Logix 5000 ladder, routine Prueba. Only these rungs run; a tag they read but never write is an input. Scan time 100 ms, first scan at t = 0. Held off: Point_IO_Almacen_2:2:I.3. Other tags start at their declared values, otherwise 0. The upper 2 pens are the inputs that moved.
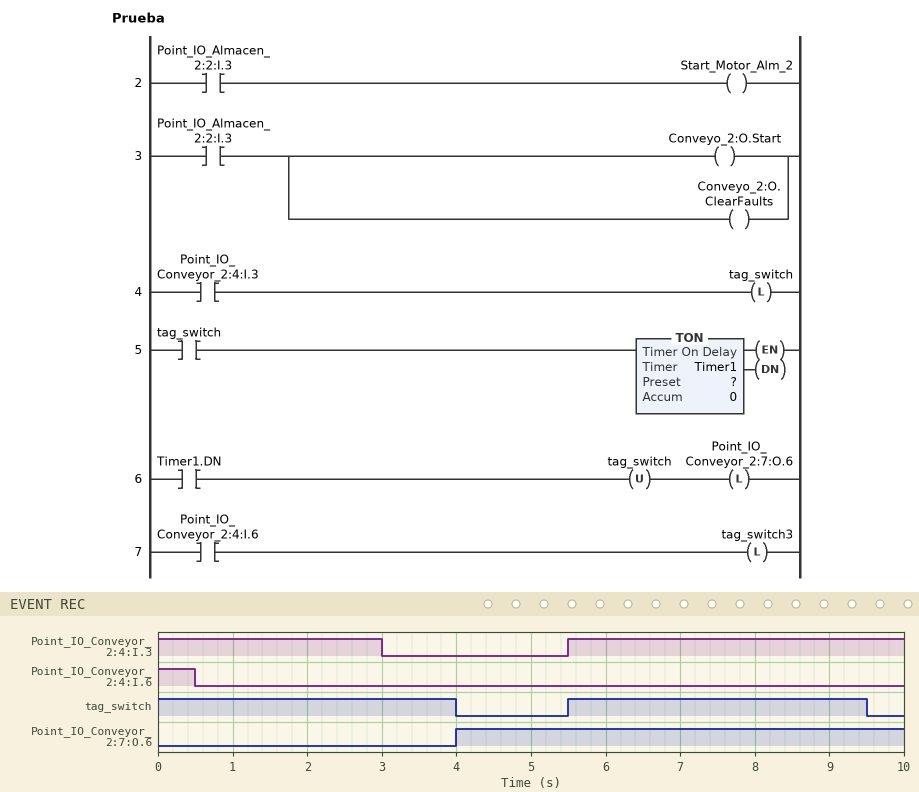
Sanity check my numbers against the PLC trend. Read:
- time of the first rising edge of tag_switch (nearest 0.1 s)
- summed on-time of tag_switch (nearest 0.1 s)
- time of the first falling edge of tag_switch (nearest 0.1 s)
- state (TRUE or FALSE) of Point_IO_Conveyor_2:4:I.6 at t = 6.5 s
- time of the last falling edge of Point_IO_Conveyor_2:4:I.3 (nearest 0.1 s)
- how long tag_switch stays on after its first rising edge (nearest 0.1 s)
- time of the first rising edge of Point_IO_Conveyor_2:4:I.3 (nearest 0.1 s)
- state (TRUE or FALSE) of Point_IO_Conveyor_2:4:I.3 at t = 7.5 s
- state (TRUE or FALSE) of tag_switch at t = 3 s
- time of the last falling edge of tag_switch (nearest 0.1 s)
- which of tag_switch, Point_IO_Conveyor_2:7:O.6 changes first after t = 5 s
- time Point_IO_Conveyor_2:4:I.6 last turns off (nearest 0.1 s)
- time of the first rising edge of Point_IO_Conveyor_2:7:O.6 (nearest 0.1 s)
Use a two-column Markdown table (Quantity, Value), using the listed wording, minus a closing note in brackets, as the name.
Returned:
| Quantity | Value |
|---|---|
| time of the first rising edge of tag_switch | 5.5 s |
| summed on-time of tag_switch | 8.0 s |
| time of the first falling edge of tag_switch | 4.0 s |
| state (TRUE or FALSE) of Point_IO_Conveyor_2:4:I.6 at t = 6.5 s | FALSE |
| time of the last falling edge of Point_IO_Conveyor_2:4:I.3 | 3.0 s |
| how long tag_switch stays on after its first rising edge | 4.0 s |
| time of the first rising edge of Point_IO_Conveyor_2:4:I.3 | 5.5 s |
| state (TRUE or FALSE) of Point_IO_Conveyor_2:4:I.3 at t = 7.5 s | TRUE |
| state (TRUE or FALSE) of tag_switch at t = 3 s | TRUE |
| time of the last falling edge of tag_switch | 9.5 s |
| which of tag_switch, Point_IO_Conveyor_2:7:O.6 changes first after t = 5 s | tag_switch |
| time Point_IO_Conveyor_2:4:I.6 last turns off | 0.5 s |
| time of the first rising edge of Point_IO_Conveyor_2:7:O.6 | 4.0 s |
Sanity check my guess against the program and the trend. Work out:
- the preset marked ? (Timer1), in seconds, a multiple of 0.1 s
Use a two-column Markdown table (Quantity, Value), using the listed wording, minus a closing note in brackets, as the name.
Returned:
| Quantity | Value |
|---|---|
| the preset marked ? (Timer1), in seconds, a multiple of 0.1 s | 4.0 s |
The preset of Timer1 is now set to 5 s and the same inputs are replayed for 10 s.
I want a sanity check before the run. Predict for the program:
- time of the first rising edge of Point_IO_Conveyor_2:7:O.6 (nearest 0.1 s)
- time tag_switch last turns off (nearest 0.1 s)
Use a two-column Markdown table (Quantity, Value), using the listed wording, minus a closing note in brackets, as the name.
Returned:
| Quantity | Value |
|---|---|
| time of the first rising edge of Point_IO_Conveyor_2:7:O.6 | 5.0 s |
| time tag_switch last turns off | 5.0 s |
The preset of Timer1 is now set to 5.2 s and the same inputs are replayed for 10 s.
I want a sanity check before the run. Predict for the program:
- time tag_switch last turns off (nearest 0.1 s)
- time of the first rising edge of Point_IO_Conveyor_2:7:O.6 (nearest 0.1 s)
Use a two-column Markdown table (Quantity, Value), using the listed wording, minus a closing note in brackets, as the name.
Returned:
| Quantity | Value |
|---|---|
| time tag_switch last turns off | 5.2 s |
| time of the first rising edge of Point_IO_Conveyor_2:7:O.6 | 5.2 s |
